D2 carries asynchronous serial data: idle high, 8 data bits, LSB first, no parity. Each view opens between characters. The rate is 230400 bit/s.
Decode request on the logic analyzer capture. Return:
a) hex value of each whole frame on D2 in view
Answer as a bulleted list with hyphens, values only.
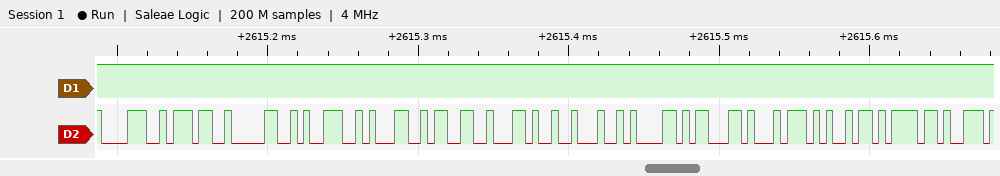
- 38, 37, 30, 39, 31, 33, 2C, 22, 61, 63, 74, 69, 6F
